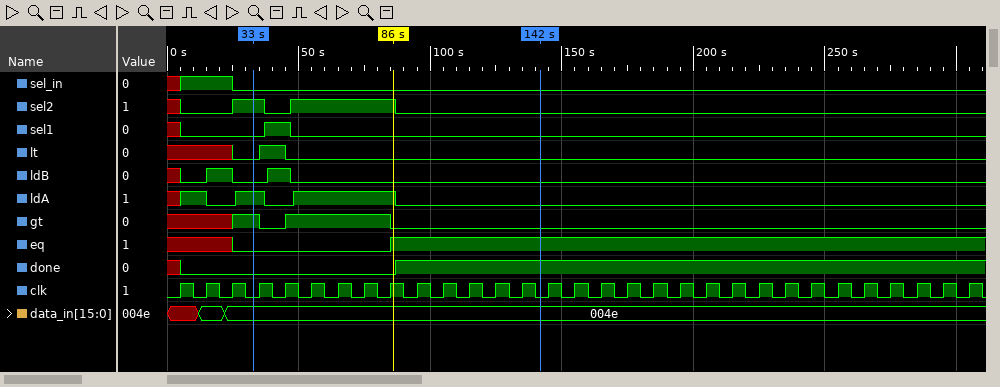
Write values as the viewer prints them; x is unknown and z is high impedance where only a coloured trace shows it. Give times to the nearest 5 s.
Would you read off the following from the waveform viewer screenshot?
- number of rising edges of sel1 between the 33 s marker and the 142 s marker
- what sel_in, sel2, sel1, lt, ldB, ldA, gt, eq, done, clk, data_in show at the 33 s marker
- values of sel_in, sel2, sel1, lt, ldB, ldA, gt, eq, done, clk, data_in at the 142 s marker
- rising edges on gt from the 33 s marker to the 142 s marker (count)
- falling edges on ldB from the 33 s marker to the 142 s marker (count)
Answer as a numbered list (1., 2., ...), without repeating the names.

1. 1
2. sel_in=0, sel2=1, sel1=0, lt=0, ldB=0, ldA=1, gt=1, eq=0, done=0, clk=0, data_in=004e
3. sel_in=0, sel2=0, sel1=0, lt=0, ldB=0, ldA=0, gt=0, eq=1, done=1, clk=0, data_in=004e
4. 1
5. 1
